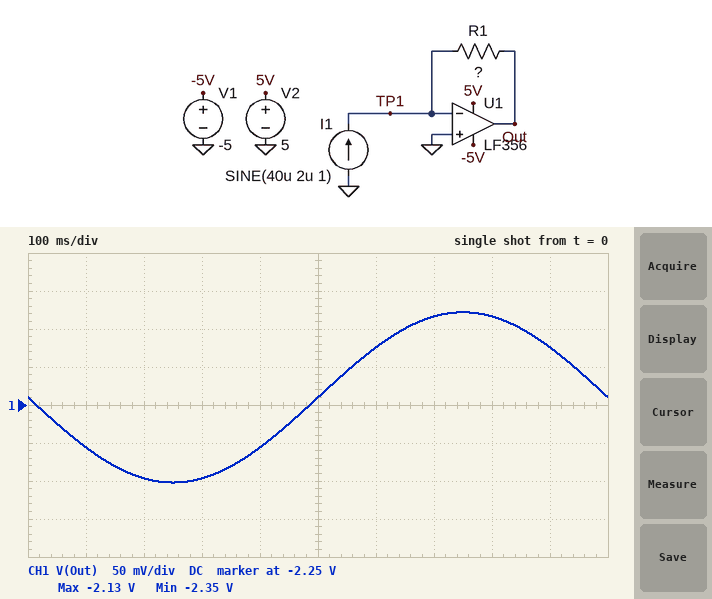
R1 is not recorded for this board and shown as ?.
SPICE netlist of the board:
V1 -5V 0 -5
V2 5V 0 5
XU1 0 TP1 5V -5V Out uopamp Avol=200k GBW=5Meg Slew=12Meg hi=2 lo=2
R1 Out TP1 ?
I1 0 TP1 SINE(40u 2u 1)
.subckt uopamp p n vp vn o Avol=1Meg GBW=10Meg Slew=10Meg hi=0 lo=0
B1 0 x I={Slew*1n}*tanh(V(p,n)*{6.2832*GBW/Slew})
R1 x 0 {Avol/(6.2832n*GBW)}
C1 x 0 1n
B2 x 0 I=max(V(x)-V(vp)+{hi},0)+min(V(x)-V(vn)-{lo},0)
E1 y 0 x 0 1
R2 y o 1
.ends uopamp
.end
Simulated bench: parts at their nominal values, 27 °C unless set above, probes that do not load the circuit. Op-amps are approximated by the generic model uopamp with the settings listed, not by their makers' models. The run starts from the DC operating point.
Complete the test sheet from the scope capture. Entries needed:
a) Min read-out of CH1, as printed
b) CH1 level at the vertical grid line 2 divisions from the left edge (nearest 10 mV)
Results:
-2.35 V
-2.35 V
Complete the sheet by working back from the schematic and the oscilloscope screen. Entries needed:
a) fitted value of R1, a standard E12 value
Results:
56 kΩ
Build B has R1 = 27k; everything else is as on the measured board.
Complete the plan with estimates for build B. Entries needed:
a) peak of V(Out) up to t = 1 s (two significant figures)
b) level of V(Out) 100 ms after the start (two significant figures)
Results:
-1.0 V
-1.1 V
